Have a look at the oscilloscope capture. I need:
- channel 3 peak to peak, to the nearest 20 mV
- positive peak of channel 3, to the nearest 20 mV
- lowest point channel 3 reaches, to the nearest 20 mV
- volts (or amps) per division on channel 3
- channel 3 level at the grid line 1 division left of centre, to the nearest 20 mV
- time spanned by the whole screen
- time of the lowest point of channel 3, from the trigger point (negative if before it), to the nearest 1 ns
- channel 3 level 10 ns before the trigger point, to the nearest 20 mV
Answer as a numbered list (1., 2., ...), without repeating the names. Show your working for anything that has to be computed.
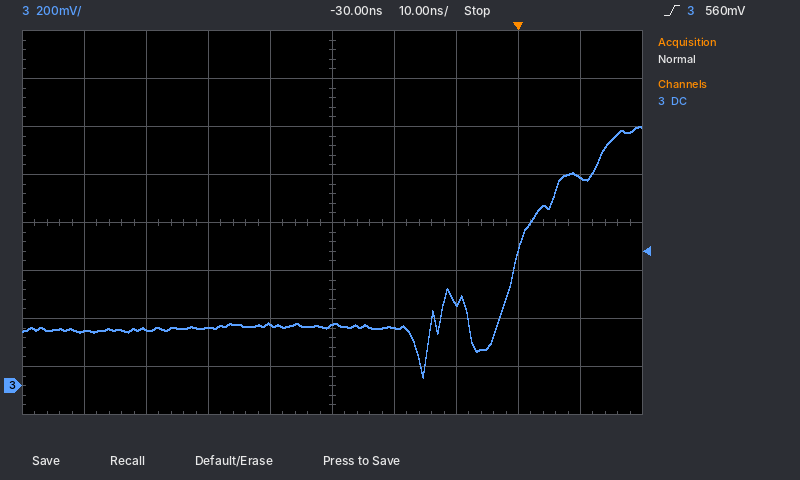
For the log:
1. 1.08 V − (40 mV) = 1.04 V
2. 1.08 V
3. 40 mV
4. 200 mV
5. 260 mV
6. 100 ns
7. -15 ns
8. 340 mV
